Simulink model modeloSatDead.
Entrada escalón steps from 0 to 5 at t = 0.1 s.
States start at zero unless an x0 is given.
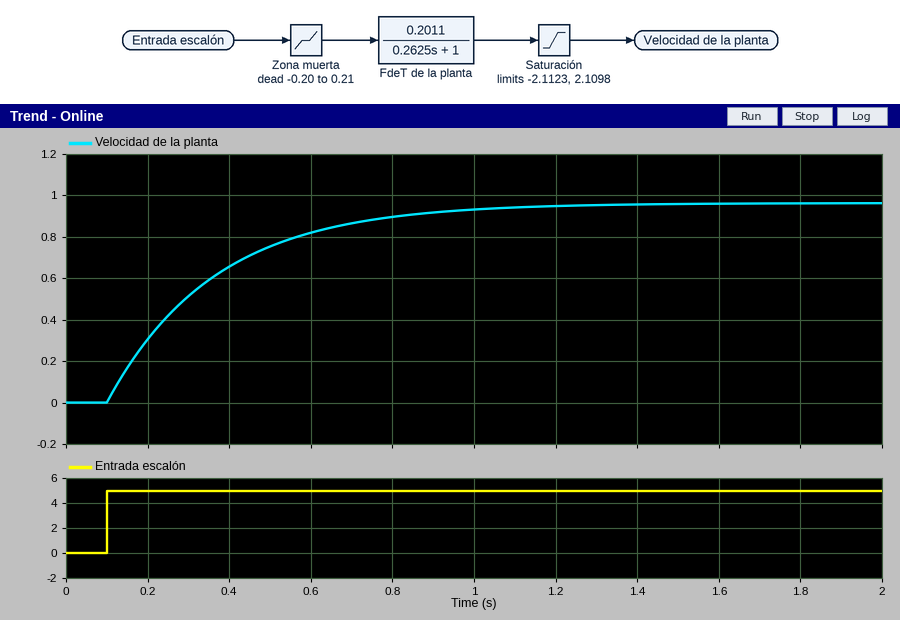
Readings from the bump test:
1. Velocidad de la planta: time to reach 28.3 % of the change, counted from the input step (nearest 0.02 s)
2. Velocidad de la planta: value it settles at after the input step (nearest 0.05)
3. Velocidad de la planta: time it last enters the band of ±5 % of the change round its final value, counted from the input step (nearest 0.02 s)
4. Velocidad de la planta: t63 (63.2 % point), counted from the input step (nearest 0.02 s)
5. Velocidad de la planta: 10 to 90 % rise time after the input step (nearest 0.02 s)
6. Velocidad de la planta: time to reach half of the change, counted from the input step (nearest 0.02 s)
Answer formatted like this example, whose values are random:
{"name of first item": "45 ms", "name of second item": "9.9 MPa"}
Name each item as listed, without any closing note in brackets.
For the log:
{"Velocidad de la planta: time to reach 28.3 % of the change, counted from the input step": "0.08 s", "Velocidad de la planta: value it settles at after the input step": "0.95", "Velocidad de la planta: time it last enters the band of ±5 % of the change round its final value, counted from the input step": "0.78 s", "Velocidad de la planta: t63 (63.2 % point), counted from the input step": "0.26 s", "Velocidad de la planta: 10 to 90 % rise time after the input step": "0.58 s", "Velocidad de la planta: time to reach half of the change, counted from the input step": "0.18 s"}
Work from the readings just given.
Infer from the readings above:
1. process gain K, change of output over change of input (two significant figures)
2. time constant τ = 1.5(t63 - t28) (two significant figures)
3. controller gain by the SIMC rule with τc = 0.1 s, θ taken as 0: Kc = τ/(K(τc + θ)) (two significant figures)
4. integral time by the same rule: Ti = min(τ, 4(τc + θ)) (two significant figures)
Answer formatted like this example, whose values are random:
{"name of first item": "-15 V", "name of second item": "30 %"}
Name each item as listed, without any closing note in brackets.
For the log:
{"process gain K, change of output over change of input": "0.19", "time constant τ = 1.5(t63 - t28)": "0.27 s", "controller gain by the SIMC rule with τc = 0.1 s, θ taken as 0: Kc = τ/(K(τc + θ))": "14", "integral time by the same rule: Ti = min(τ, 4(τc + θ))": "0.27 s"}
